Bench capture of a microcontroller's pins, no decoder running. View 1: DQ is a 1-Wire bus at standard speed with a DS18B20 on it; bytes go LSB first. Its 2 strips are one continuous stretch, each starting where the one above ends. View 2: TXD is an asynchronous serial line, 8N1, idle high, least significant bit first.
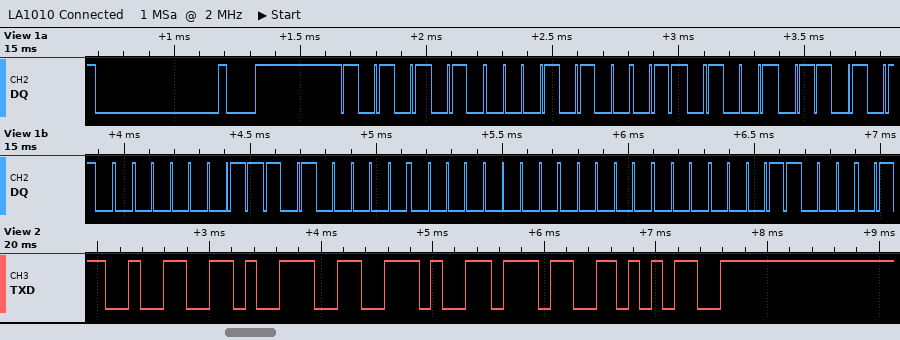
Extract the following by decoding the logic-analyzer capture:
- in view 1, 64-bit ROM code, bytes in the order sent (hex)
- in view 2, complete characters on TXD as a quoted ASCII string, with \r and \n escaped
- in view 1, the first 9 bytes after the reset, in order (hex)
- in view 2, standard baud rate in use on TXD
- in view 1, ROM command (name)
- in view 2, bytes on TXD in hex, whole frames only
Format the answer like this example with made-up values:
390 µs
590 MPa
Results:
28 96 56 C0 05 00 00 18
"29.75"
55 28 96 56 C0 05 00 00 18
9600 baud
Match ROM
0x32 0x39 0x2E 0x37 0x35
